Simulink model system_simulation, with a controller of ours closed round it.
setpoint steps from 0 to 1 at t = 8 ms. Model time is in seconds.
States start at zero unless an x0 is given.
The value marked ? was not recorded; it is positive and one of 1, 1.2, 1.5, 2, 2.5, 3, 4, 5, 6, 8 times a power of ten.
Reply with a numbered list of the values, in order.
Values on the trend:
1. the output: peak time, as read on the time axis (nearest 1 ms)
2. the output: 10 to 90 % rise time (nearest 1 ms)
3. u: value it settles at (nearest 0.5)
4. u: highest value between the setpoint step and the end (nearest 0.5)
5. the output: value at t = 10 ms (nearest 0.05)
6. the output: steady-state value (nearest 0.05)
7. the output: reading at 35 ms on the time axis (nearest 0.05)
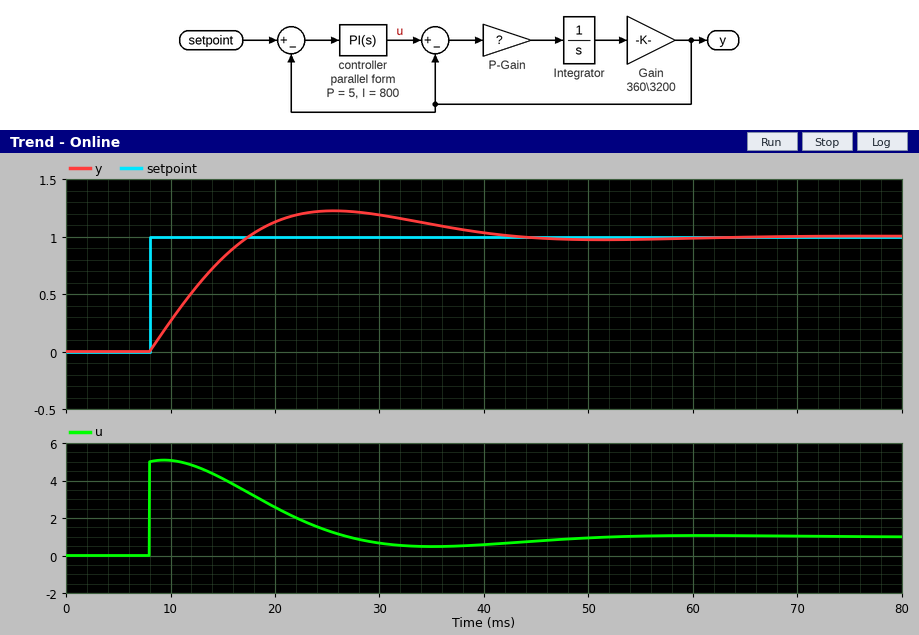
1. 26 ms
2. 7 ms
3. 1.0
4. 5.0
5. 0.25
6. 1.00
7. 1.10
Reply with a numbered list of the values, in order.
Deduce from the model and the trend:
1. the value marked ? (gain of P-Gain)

1. 3
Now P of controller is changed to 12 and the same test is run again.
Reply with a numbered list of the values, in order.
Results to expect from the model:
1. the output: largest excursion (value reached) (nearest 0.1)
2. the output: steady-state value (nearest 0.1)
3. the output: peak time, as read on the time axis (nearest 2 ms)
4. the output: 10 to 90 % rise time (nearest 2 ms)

1. 1.1
2. 1.0
3. 22 ms
4. 6 ms
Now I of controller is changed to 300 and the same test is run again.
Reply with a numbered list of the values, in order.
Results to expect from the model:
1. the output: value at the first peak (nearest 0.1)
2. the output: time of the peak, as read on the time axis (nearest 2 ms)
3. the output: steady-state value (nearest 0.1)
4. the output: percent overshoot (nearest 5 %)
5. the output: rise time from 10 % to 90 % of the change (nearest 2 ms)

1. 1.1
2. 36 ms
3. 1.0
4. 10 %
5. 12 ms
